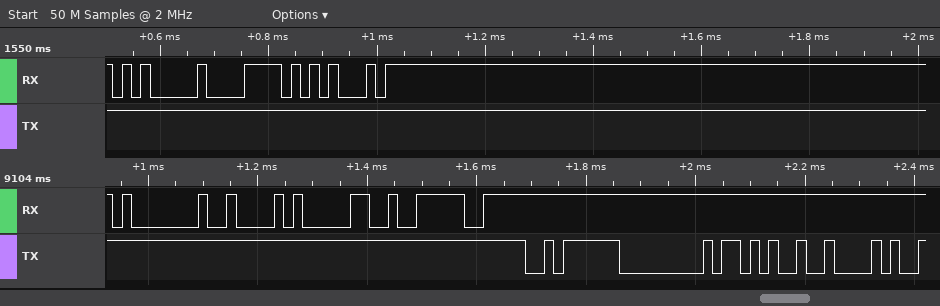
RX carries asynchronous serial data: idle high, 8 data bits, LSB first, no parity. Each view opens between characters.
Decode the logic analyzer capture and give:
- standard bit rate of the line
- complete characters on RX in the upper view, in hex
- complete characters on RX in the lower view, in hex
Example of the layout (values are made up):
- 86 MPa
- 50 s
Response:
- 57600 baud
- 05, 78, 45
- 01, 42, 30, 3E
